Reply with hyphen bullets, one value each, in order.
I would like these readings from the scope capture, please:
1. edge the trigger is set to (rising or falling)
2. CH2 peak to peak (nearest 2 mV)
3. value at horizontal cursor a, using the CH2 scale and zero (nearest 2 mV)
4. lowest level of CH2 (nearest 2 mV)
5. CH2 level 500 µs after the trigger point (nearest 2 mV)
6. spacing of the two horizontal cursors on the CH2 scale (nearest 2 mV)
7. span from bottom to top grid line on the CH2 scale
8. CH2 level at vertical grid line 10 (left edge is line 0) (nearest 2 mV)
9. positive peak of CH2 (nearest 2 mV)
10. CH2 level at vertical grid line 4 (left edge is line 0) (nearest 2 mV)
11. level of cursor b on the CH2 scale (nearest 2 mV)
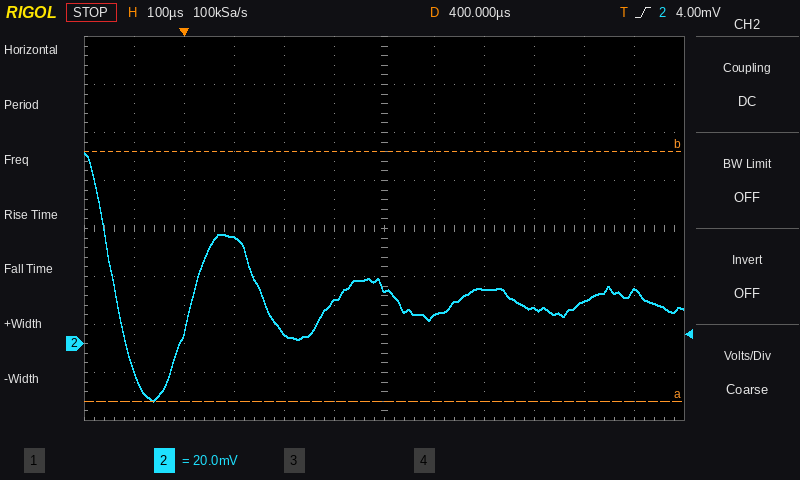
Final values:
- rising
- 104 mV
- -24 mV
- -24 mV
- 12 mV
- 104 mV
- 160 mV
- 18 mV
- 80 mV
- 4 mV
- 80 mV
